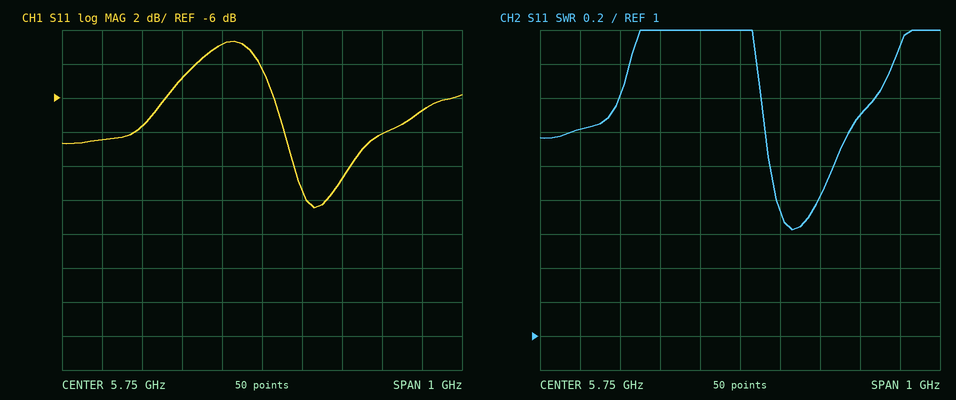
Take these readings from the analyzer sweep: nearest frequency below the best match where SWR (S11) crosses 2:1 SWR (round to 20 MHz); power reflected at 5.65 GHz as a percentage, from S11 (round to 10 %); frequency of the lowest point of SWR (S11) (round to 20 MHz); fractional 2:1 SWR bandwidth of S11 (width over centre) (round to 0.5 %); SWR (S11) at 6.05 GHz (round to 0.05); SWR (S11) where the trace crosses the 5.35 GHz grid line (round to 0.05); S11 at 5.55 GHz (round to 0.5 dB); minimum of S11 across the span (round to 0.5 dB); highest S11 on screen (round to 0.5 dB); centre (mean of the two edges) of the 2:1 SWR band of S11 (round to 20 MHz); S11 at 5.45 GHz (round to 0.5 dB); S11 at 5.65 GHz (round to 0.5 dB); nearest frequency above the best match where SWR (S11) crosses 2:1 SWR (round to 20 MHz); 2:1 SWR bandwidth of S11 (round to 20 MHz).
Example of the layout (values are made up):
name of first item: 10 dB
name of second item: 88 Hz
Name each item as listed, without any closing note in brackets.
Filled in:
nearest frequency below the best match where SWR (S11) crosses 2:1 SWR: 5.82 GHz
power reflected at 5.65 GHz as a percentage, from S11: 50 %
frequency of the lowest point of SWR (S11): 5.88 GHz
fractional 2:1 SWR bandwidth of S11 (width over centre): 2.5 %
SWR (S11) at 6.05 GHz: 2.30
SWR (S11) where the trace crosses the 5.35 GHz grid line: 2.20
S11 at 5.55 GHz: -5.0 dB
minimum of S11 across the span: -12.5 dB
highest S11 on screen: -2.5 dB
centre (mean of the two edges) of the 2:1 SWR band of S11: 5.90 GHz
S11 at 5.45 GHz: -7.5 dB
S11 at 5.65 GHz: -3.0 dB
nearest frequency above the best match where SWR (S11) crosses 2:1 SWR: 5.98 GHz
2:1 SWR bandwidth of S11: 160 MHz
